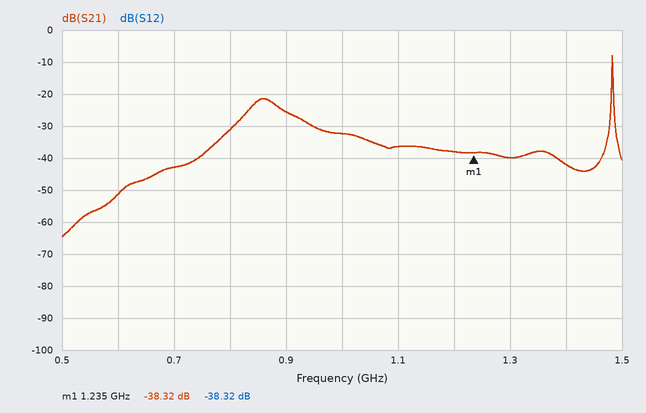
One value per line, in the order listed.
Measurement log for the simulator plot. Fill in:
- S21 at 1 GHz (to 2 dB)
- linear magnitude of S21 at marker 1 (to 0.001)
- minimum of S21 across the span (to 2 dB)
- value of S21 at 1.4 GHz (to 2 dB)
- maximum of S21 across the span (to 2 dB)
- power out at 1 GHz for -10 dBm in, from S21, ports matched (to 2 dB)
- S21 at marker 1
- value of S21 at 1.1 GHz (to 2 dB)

-32 dB
0.012
-64 dB
-42 dB
-8 dB
-42 dBm
-38.32 dB
-36 dB
